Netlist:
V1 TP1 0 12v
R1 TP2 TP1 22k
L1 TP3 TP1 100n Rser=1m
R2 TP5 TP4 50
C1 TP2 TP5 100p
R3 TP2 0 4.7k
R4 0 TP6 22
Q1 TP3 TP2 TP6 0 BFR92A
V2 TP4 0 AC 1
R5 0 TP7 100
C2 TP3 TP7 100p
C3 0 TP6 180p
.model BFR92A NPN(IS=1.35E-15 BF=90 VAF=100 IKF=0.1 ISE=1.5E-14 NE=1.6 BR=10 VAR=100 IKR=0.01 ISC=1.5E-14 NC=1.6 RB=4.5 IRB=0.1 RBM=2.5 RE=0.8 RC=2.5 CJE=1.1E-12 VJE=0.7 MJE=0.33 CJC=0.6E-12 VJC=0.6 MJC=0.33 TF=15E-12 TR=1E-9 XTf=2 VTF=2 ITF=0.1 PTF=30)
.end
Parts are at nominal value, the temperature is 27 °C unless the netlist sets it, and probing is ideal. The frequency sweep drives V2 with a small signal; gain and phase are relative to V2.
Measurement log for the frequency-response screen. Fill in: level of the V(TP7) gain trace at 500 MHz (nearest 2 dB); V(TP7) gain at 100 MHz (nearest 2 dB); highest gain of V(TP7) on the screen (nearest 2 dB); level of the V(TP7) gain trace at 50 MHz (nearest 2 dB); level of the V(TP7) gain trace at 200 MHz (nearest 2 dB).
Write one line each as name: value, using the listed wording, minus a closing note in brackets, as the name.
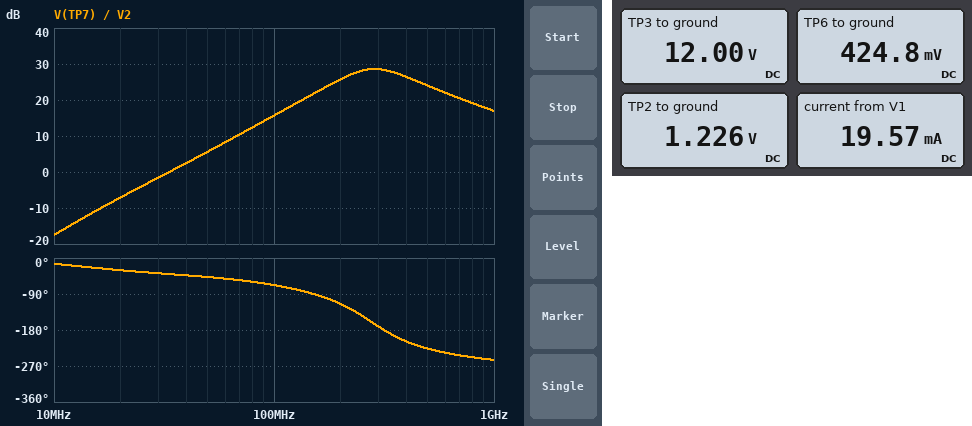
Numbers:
level of the V(TP7) gain trace at 500 MHz: 24 dB
V(TP7) gain at 100 MHz: 16 dB
highest gain of V(TP7) on the screen: 28 dB
level of the V(TP7) gain trace at 50 MHz: 6 dB
level of the V(TP7) gain trace at 200 MHz: 26 dB
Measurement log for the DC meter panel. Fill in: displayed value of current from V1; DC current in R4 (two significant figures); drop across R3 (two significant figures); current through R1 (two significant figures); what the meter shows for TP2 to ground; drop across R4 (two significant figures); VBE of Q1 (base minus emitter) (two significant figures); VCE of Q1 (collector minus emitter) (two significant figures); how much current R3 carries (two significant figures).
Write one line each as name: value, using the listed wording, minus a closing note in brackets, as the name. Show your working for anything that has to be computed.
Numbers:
displayed value of current from V1: 19.57 mA
DC current in R4: (424.8 mV) / 22 Ω = 19 mA
drop across R3: 1.226 V = 1.2 V
current through R1: (12 V - 1.226 V) / 22 kΩ = 490 µA
what the meter shows for TP2 to ground: 1.226 V
drop across R4: 424.8 mV = 420 mV
VBE of Q1 (base minus emitter): 1.226 V - 424.8 mV = 800 mV
VCE of Q1 (collector minus emitter): 12 V - 424.8 mV = 12 V
how much current R3 carries: (1.226 V) / 4.7 kΩ = 260 µA
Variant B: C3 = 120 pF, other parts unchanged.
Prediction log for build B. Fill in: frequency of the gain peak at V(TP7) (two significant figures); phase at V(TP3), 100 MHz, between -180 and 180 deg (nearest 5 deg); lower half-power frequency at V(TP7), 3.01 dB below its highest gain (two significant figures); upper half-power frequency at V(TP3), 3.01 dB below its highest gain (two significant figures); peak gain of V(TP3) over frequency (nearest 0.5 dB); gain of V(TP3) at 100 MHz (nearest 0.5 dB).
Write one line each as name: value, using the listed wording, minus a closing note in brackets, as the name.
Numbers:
frequency of the gain peak at V(TP7): 340 MHz
phase at V(TP3), 100 MHz, between -180 and 180 deg: -80 deg
lower half-power frequency at V(TP7), 3.01 dB below its highest gain: 240 MHz
upper half-power frequency at V(TP3), 3.01 dB below its highest gain: 490 MHz
peak gain of V(TP3) over frequency: 28.0 dB
gain of V(TP3) at 100 MHz: 13.0 dB
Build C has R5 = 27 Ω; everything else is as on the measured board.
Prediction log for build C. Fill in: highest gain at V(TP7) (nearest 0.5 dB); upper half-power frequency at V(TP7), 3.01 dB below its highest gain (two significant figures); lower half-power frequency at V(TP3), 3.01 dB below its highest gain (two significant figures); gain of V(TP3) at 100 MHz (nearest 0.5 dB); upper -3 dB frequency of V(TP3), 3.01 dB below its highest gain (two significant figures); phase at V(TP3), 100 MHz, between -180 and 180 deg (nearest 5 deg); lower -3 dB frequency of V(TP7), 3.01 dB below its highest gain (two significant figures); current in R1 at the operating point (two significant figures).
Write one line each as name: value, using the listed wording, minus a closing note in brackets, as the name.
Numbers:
highest gain at V(TP7): 17.0 dB
upper half-power frequency at V(TP7), 3.01 dB below its highest gain: 630 MHz
lower half-power frequency at V(TP3), 3.01 dB below its highest gain: 170 MHz
gain of V(TP3) at 100 MHz: 11.5 dB
upper -3 dB frequency of V(TP3), 3.01 dB below its highest gain: 620 MHz
phase at V(TP3), 100 MHz, between -180 and 180 deg: -135 deg
lower -3 dB frequency of V(TP7), 3.01 dB below its highest gain: 180 MHz
current in R1 at the operating point: 490 µA
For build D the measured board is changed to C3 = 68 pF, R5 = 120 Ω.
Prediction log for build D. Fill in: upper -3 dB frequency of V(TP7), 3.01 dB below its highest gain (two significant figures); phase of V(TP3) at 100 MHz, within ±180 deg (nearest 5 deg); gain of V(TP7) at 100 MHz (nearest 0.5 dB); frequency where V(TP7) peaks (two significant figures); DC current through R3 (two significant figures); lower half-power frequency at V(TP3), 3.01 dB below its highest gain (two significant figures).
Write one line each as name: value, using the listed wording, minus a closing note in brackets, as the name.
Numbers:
upper -3 dB frequency of V(TP7), 3.01 dB below its highest gain: 570 MHz
phase of V(TP3) at 100 MHz, within ±180 deg: -85 deg
gain of V(TP7) at 100 MHz: 10.0 dB
frequency where V(TP7) peaks: 420 MHz
DC current through R3: 260 µA
lower half-power frequency at V(TP3), 3.01 dB below its highest gain: 310 MHz
